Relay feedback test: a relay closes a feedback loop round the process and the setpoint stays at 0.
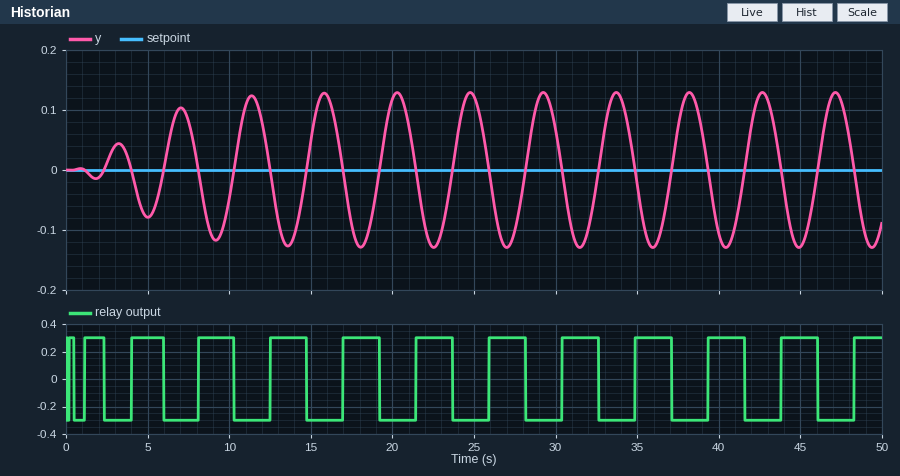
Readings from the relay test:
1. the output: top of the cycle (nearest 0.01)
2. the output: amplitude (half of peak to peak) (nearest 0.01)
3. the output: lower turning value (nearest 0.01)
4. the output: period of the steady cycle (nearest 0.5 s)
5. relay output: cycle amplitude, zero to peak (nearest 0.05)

0.13
0.13
-0.13
4.5 s
0.30
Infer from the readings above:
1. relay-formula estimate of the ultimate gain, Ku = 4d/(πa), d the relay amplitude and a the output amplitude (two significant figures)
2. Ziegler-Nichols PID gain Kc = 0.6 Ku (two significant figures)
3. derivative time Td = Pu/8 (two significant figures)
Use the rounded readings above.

2.9
1.7
0.56 s
